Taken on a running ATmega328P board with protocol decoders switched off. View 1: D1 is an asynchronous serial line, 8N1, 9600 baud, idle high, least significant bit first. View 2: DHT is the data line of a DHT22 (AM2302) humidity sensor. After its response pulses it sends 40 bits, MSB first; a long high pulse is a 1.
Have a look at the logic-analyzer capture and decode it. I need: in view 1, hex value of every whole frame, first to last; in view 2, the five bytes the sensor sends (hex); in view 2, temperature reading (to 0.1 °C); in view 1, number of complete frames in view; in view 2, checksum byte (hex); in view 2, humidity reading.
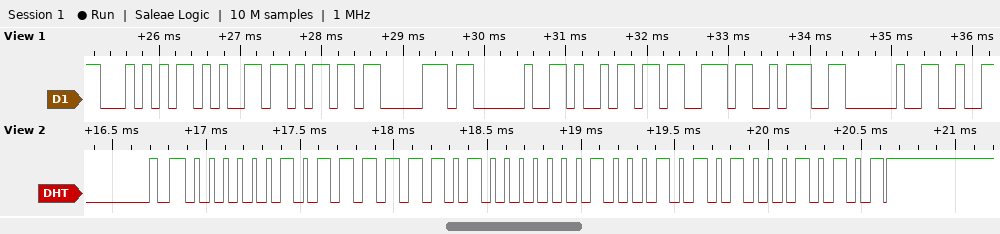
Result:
54 65 6D 70 20 69 73 3A 20
02 FD 01 15 15
27.7 °C
9
0x15
76.5 %
